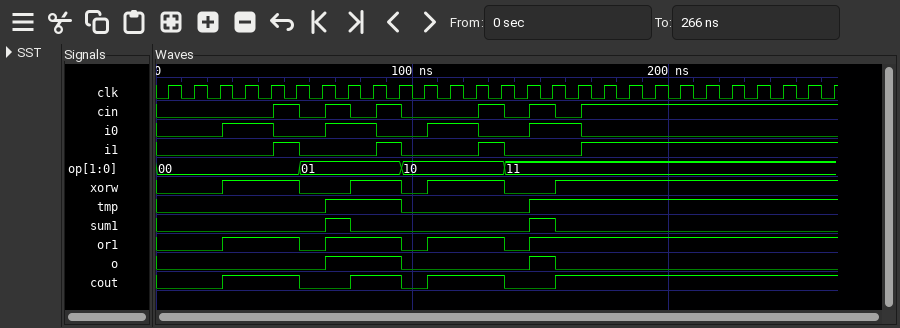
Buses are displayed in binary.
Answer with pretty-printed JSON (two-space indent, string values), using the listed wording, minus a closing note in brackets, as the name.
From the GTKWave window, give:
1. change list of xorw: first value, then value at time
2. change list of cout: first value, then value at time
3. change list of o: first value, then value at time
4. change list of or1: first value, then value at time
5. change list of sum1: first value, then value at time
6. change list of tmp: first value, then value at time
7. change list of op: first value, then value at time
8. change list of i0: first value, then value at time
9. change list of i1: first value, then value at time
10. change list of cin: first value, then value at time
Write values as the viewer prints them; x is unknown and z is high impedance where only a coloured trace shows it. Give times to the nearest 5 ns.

{
  "change list of xorw: first value, then value at time": "0, 1 at 25 ns, 0 at 55 ns, 1 at 75 ns, 0 at 95 ns, 1 at 105 ns, 0 at 135 ns, 1 at 155 ns",
  "change list of cout: first value, then value at time": "0, 1 at 25 ns, 0 at 55 ns, 1 at 75 ns, 0 at 95 ns, 1 at 105 ns, 0 at 135 ns, 1 at 155 ns",
  "change list of o: first value, then value at time": "0, 1 at 65 ns, 0 at 95 ns, 1 at 145 ns, 0 at 155 ns",
  "change list of or1: first value, then value at time": "0, 1 at 25 ns, 0 at 55 ns, 1 at 65 ns, 0 at 95 ns, 1 at 105 ns, 0 at 135 ns, 1 at 145 ns",
  "change list of sum1: first value, then value at time": "0, 1 at 65 ns, 0 at 75 ns, 1 at 145 ns, 0 at 155 ns",
  "change list of tmp: first value, then value at time": "0, 1 at 65 ns, 0 at 95 ns, 1 at 145 ns",
  "change list of op: first value, then value at time": "00, 01 at 55 ns, 10 at 95 ns, 11 at 135 ns",
  "change list of i0: first value, then value at time": "0, 1 at 25 ns, 0 at 45 ns, 1 at 65 ns, 0 at 85 ns, 1 at 105 ns, 0 at 125 ns, 1 at 145 ns, 0 at 165 ns",
  "change list of i1: first value, then value at time": "0, 1 at 45 ns, 0 at 55 ns, 1 at 85 ns, 0 at 95 ns, 1 at 125 ns, 0 at 135 ns, 1 at 165 ns",
  "change list of cin: first value, then value at time": "0, 1 at 45 ns, 0 at 55 ns, 1 at 65 ns, 0 at 75 ns, 1 at 85 ns, 0 at 95 ns, 1 at 125 ns, 0 at 135 ns, 1 at 145 ns, 0 at 155 ns, 1 at 165 ns"
}
